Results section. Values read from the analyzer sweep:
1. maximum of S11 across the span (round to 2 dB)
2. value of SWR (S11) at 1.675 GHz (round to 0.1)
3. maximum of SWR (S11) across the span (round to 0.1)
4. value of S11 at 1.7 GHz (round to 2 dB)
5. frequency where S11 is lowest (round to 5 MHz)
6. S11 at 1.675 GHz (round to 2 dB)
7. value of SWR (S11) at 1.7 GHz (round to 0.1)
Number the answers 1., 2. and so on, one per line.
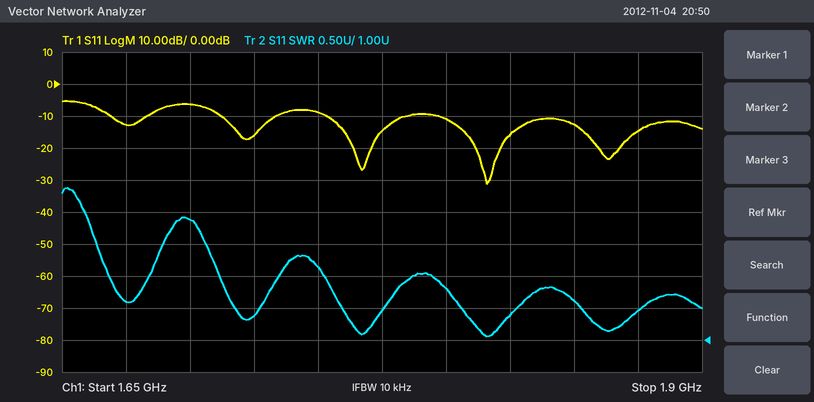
1. -6 dB
2. 1.6
3. 3.4
4. -6 dB
5. 1.815 GHz
6. -12 dB
7. 2.9
